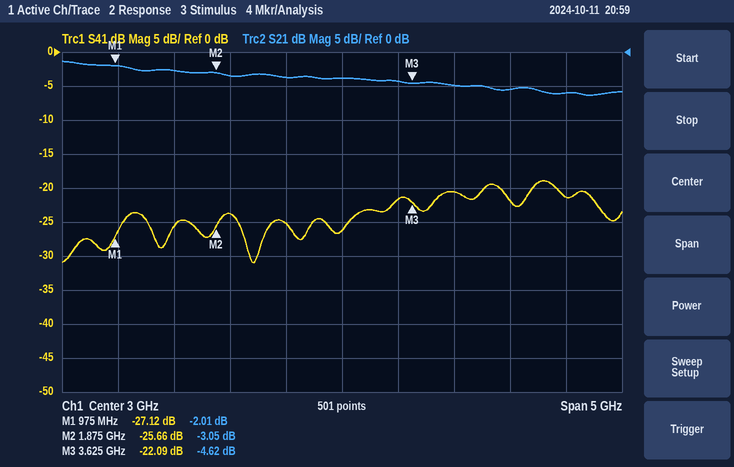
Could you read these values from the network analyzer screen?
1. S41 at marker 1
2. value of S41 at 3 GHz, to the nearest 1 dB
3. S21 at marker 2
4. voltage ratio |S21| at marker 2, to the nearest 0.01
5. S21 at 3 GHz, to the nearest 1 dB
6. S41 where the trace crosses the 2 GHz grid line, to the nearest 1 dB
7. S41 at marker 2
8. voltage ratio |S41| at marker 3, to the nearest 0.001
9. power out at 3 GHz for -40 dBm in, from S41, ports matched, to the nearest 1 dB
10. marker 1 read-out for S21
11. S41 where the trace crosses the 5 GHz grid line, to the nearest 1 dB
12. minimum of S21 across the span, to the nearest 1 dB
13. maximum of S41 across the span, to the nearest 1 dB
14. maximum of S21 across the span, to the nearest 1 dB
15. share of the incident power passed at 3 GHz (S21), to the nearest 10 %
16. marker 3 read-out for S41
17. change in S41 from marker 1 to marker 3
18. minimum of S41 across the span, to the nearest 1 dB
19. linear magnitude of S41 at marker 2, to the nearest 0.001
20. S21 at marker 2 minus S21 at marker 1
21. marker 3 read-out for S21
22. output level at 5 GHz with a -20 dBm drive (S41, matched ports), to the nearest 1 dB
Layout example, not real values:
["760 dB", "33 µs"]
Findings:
["-27.12 dB", "-26 dB", "-3.05 dB", "0.70", "-4 dB", "-24 dB", "-25.66 dB", "0.079", "-66 dBm", "-2.01 dB", "-21 dB", "-6 dB", "-19 dB", "-1 dB", "40 %", "-22.09 dB", "5.03 dB", "-31 dB", "0.052", "-1.04 dB", "-4.62 dB", "-41 dBm"]
